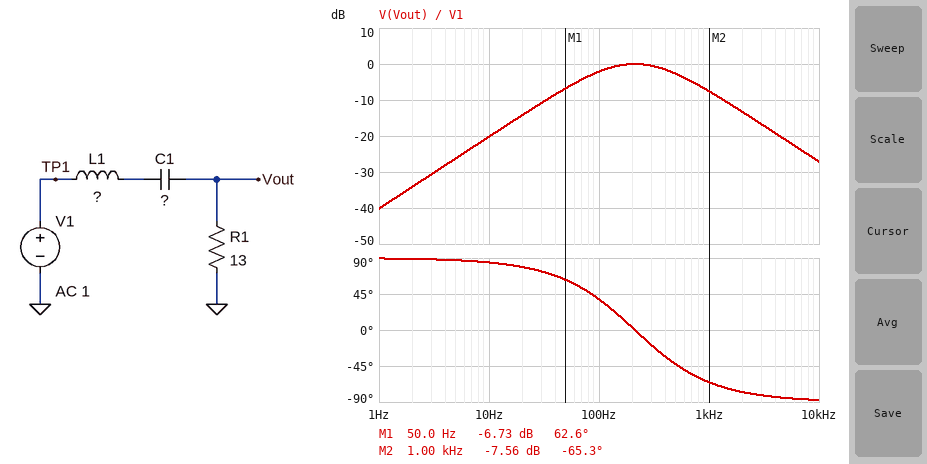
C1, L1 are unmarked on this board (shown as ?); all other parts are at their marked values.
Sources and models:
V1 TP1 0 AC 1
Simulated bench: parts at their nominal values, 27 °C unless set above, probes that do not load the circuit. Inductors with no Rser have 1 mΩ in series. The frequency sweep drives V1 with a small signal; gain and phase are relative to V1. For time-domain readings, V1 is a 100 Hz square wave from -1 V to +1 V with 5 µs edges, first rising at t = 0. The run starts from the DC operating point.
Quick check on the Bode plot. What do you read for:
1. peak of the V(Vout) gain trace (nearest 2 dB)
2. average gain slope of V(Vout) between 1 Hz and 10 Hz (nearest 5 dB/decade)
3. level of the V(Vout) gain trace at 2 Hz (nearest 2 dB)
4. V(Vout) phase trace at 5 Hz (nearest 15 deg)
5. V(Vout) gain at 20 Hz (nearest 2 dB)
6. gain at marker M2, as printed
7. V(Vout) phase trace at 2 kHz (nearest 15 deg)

0 dB
20 dB/decade
-34 dB
90 deg
-14 dB
-7.56 dB
-75 deg
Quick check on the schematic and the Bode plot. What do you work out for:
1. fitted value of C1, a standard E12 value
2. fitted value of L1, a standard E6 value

120 µF
4.7 mH
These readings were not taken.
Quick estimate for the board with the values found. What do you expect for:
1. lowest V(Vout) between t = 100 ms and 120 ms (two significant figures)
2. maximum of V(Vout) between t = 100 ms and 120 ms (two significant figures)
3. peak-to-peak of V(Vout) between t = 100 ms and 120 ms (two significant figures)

-1.5 V
1.5 V
2.9 V
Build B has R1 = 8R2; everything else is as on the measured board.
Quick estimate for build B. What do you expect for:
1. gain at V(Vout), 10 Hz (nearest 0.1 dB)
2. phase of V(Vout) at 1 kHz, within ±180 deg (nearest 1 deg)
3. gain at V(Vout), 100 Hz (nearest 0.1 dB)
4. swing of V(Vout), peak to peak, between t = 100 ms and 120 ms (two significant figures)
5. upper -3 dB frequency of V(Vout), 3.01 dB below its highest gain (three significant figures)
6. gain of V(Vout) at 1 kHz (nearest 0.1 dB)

-24.2 dB
-74 deg
-4.1 dB
2.5 V
392 Hz
-11.1 dB
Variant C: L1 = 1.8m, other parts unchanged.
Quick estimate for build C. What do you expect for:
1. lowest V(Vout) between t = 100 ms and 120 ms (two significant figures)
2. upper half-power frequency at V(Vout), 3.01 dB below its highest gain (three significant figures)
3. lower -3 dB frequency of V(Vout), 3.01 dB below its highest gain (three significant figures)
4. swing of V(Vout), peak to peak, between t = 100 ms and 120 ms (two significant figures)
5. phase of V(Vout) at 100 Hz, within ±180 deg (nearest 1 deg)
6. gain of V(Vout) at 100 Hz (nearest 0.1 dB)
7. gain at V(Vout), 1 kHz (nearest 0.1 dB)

-1.6 V
1.24 kHz
94.3 Hz
3.3 V
43 deg
-2.7 dB
-2.0 dB
